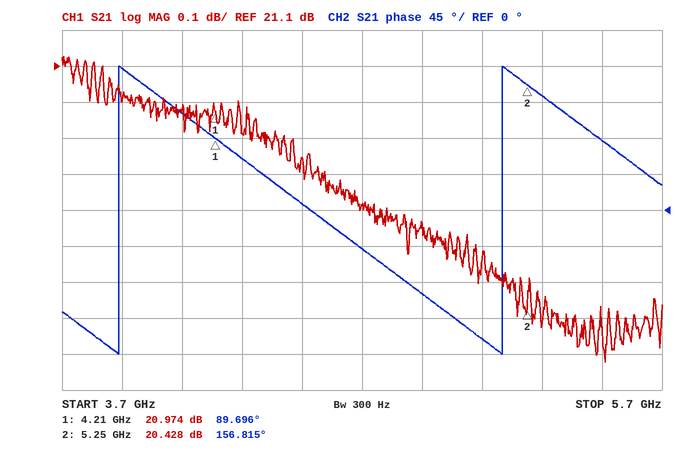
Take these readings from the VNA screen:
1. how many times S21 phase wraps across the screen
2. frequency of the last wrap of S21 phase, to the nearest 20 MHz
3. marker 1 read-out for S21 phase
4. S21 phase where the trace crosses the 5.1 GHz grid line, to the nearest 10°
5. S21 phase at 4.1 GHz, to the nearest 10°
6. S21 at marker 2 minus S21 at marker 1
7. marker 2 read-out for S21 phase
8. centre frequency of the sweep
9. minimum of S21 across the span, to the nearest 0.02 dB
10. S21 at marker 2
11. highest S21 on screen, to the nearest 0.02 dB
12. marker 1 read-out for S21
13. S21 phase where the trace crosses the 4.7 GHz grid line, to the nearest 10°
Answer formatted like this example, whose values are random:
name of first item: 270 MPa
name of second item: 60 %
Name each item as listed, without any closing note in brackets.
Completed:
how many times S21 phase wraps across the screen: 2
frequency of the last wrap of S21 phase, to the nearest 20 MHz: 5.16 GHz
marker 1 read-out for S21 phase: 89.696°
S21 phase where the trace crosses the 5.1 GHz grid line, to the nearest 10°: -160°
S21 phase at 4.1 GHz, to the nearest 10°: 120°
S21 at marker 2 minus S21 at marker 1: -0.546 dB
marker 2 read-out for S21 phase: 156.815°
centre frequency of the sweep: 4.7 GHz
minimum of S21 across the span, to the nearest 0.02 dB: 20.28 dB
S21 at marker 2: 20.428 dB
highest S21 on screen, to the nearest 0.02 dB: 21.12 dB
marker 1 read-out for S21: 20.974 dB
S21 phase where the trace crosses the 4.7 GHz grid line, to the nearest 10°: -50°
